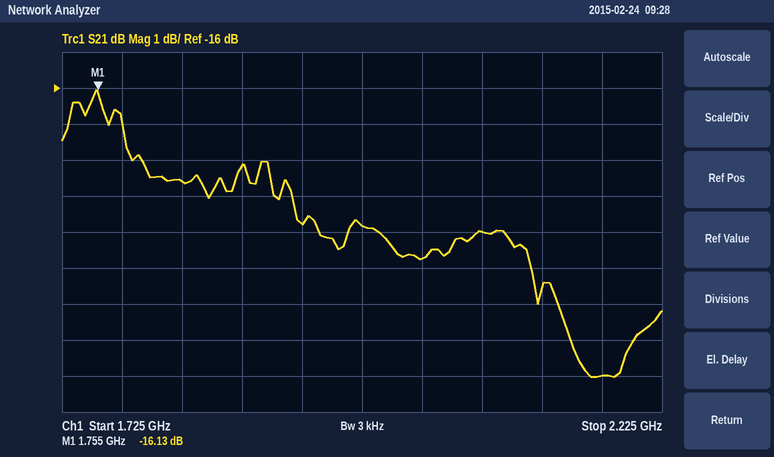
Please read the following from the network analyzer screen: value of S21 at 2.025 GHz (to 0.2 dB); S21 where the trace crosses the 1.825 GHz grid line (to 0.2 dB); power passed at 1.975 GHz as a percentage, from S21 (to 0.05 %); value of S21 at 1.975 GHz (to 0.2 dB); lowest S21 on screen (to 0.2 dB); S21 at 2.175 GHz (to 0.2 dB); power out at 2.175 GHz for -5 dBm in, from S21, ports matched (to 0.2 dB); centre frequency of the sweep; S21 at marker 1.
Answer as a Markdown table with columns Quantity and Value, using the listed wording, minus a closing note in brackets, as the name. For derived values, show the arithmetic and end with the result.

| Quantity | Value |
|---|---|
| value of S21 at 2.025 GHz | -20.8 dB |
| S21 where the trace crosses the 1.825 GHz grid line | -18.6 dB |
| power passed at 1.975 GHz as a percentage, from S21 | 10^(-19.8/10) ≈ 1.05 % |
| value of S21 at 1.975 GHz | -19.8 dB |
| lowest S21 on screen | -24.0 dB |
| S21 at 2.175 GHz | -24.0 dB |
| power out at 2.175 GHz for -5 dBm in, from S21, ports matched | -5 dBm + (-24.0 dB) = -29.0 dBm |
| centre frequency of the sweep | 1.975 GHz |
| S21 at marker 1 | -16.13 dB |
